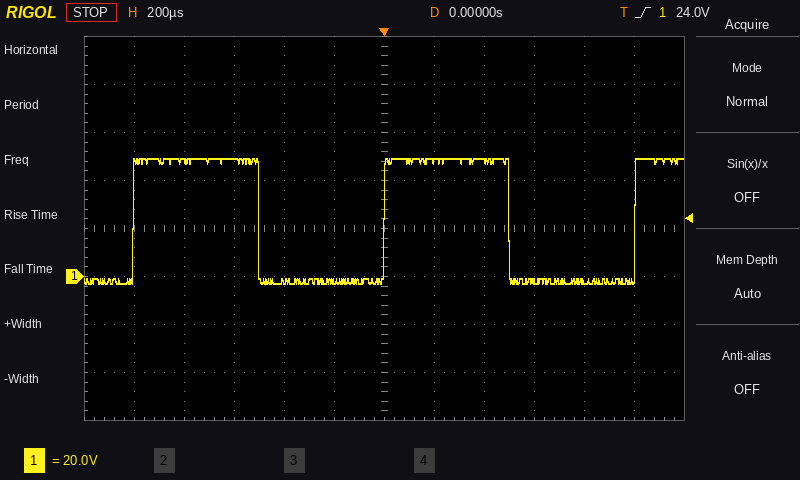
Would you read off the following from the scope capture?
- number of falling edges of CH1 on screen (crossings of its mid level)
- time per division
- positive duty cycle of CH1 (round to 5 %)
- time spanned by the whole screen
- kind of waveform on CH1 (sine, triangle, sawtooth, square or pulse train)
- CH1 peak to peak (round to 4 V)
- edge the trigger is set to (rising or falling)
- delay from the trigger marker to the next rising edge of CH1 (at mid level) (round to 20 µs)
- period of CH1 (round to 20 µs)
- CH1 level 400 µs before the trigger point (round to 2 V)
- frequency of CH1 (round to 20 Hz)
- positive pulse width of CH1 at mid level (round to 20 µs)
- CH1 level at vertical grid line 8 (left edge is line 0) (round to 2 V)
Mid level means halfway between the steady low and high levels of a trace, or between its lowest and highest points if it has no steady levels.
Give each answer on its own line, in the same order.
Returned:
2
200 µs
50 %
2.4 ms
square
52 V
rising
1.00 ms
1.00 ms
-2 V
1.00 kHz
500 µs
48 V
